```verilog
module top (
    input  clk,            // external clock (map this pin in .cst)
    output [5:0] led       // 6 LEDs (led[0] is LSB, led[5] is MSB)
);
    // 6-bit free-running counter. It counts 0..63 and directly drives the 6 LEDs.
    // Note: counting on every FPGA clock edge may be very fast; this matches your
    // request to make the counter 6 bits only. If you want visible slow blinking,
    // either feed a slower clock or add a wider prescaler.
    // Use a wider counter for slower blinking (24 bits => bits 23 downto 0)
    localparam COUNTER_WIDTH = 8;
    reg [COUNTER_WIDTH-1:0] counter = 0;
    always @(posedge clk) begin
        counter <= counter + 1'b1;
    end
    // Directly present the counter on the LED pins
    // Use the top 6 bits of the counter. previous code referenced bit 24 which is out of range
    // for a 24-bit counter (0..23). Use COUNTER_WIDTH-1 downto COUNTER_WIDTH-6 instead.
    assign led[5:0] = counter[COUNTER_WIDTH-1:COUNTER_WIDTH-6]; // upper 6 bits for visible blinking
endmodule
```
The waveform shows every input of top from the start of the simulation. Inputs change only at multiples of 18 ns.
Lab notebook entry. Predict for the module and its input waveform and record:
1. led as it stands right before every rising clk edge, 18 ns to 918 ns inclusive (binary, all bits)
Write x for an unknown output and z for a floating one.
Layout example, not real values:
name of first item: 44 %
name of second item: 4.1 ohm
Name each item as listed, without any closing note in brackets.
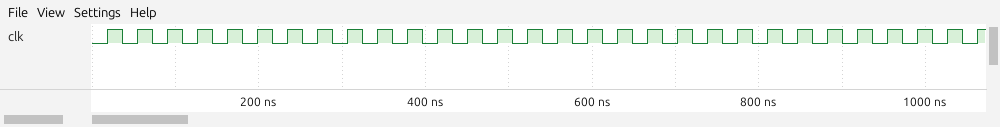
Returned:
led as it stands right before every rising clk edge, 18 ns to 918 ns inclusive: 000000, 000000, 000000, 000000, 000001, 000001, 000001, 000001, 000010, 000010, 000010, 000010, 000011, 000011, 000011, 000011, 000100, 000100, 000100, 000100, 000101, 000101, 000101, 000101, 000110, 000110
